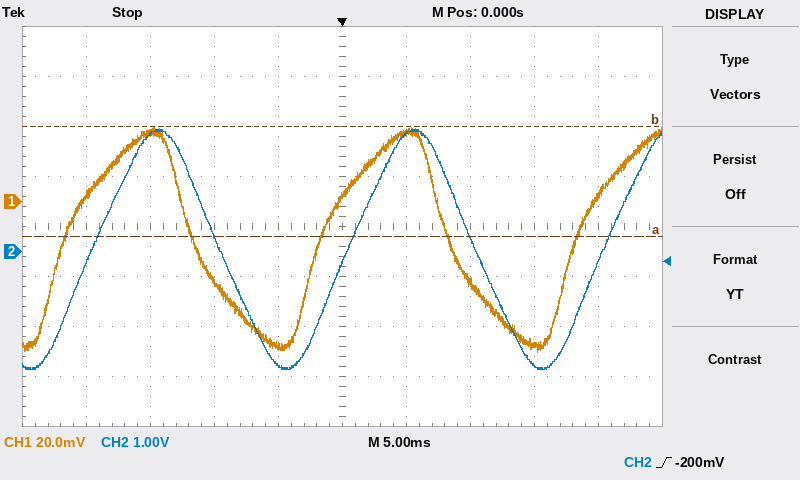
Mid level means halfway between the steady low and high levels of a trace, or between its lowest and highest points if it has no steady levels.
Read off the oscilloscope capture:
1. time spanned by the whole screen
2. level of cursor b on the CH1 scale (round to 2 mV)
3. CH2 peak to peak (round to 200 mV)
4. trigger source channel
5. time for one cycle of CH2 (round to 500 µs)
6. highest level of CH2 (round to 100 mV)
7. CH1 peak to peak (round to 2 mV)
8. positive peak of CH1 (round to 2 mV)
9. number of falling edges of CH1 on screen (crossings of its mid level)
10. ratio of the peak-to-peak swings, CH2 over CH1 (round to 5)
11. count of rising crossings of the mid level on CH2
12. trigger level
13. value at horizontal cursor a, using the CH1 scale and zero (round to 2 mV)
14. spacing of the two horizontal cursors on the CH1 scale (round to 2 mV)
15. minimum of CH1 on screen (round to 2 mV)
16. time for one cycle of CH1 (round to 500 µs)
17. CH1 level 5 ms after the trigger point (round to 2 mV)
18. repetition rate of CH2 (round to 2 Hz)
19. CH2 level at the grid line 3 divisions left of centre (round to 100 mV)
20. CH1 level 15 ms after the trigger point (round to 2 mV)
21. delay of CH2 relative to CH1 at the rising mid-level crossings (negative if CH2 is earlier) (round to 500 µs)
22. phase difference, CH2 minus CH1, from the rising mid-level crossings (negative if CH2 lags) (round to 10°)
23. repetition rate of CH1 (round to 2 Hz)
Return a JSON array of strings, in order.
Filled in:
["50 ms", "30 mV", "4.8 V", "CH2", "20.0 ms", "2.4 V", "90 mV", "30 mV", "2", "55", "3", "-200 mV", "-14 mV", "44 mV", "-60 mV", "20.0 ms", "28 mV", "50 Hz", "2.3 V", "-58 mV", "+2.0 ms", "-40°", "50 Hz"]
